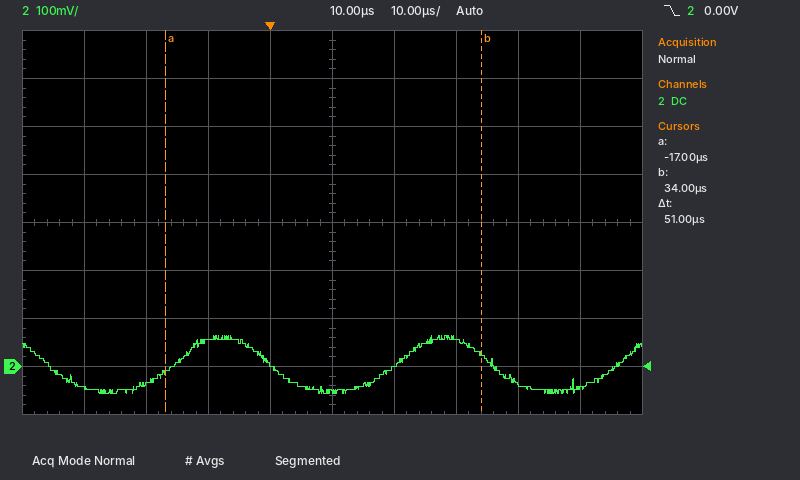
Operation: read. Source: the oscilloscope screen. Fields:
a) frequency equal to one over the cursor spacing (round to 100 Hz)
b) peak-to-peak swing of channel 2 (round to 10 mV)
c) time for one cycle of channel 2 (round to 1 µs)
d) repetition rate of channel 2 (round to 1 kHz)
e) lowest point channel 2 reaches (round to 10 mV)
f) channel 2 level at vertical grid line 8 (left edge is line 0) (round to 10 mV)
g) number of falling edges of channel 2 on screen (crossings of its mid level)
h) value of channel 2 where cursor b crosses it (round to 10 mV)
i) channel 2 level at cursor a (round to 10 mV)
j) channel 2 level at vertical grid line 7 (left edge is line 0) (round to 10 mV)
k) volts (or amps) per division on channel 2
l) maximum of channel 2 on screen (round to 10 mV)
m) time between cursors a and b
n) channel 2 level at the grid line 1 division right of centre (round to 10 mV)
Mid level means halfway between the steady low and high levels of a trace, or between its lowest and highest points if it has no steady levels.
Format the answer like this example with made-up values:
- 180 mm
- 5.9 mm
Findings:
- 19.6 kHz
- 120 mV
- 36 µs
- 28 kHz
- -60 mV
- -40 mV
- 3
- 20 mV
- -10 mV
- 60 mV
- 100 mV
- 60 mV
- 51 µs
- 0 mV
